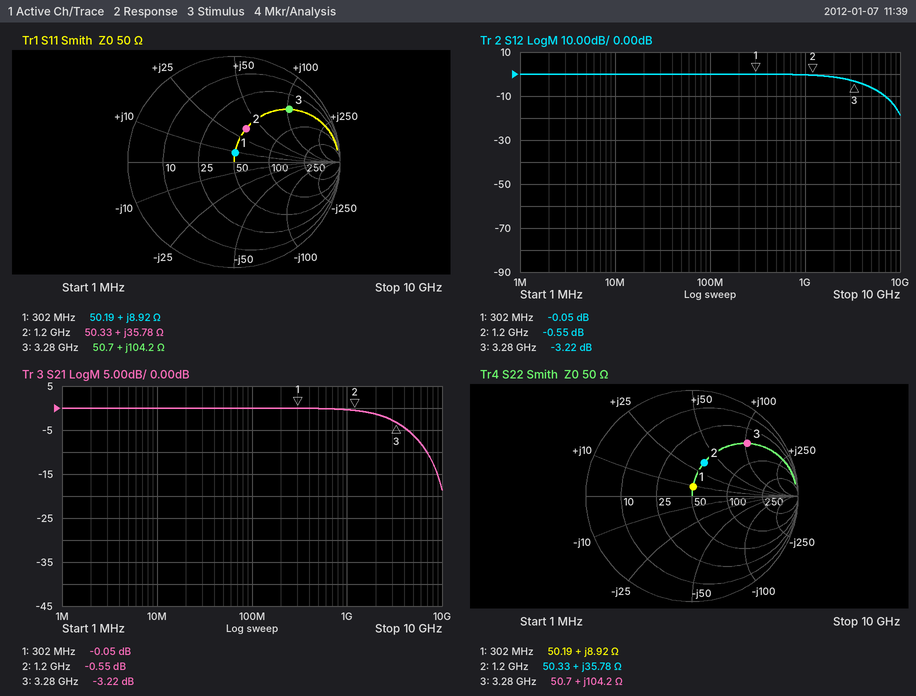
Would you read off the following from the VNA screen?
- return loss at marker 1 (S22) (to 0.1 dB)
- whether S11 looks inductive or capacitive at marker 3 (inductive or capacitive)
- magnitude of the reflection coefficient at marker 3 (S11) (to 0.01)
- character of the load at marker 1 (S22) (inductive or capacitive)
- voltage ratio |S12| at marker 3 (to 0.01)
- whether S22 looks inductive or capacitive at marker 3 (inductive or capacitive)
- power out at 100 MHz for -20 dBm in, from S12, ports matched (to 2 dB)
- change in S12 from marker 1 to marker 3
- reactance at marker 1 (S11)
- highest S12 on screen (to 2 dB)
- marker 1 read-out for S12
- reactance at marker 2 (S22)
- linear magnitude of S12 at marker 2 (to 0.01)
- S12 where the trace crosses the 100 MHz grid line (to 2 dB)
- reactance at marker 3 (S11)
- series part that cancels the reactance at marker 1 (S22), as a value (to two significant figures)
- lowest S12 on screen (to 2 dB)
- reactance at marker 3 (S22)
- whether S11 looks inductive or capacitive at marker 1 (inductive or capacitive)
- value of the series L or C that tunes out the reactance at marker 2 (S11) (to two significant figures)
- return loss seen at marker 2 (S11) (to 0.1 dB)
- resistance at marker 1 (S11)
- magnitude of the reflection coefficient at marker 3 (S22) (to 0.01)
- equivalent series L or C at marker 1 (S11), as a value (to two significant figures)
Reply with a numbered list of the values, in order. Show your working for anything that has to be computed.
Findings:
1. 21.0 dB
2. inductive
3. 0.72
4. inductive
5. 10^(-3.22/20) ≈ 0.69
6. inductive
7. -20 dBm + (0 dB) = -20 dBm
8. -3.22 − (-0.05) = -3.17 dB
9. +8.92 Ω
10. 0 dB
11. -0.05 dB
12. +35.78 Ω
13. 10^(-0.55/20) ≈ 0.94
14. 0 dB
15. +104.2 Ω
16. C = 1/(2π × 302 MHz × 8.92 Ω) ≈ 59 pF
17. -18 dB
18. +104.2 Ω
19. inductive
20. C = 1/(2π × 1.2 GHz × 35.78 Ω) ≈ 3.7 pF
21. 9.5 dB
22. 50.19 Ω
23. 0.72
24. L = 8.92 Ω/(2π × 302 MHz) ≈ 4.7 nH
